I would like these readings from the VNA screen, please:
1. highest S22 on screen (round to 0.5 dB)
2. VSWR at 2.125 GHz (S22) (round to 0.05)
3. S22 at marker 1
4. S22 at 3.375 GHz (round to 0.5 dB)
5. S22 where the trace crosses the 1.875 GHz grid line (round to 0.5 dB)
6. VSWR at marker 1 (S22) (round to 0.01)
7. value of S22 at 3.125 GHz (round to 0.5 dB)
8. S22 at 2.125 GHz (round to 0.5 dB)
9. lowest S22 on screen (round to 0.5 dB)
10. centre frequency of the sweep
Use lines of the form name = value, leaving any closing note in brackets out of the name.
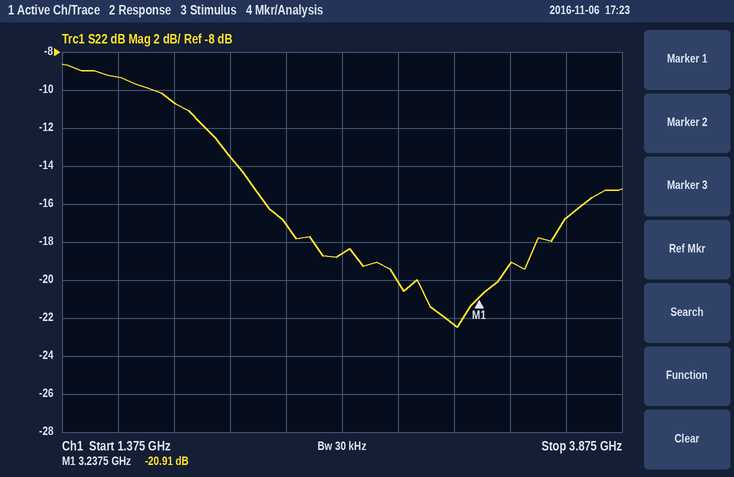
highest S22 on screen = -8.5 dB
VSWR at 2.125 GHz (S22) = 1.55
S22 at marker 1 = -20.91 dB
S22 at 3.375 GHz = -19.0 dB
S22 where the trace crosses the 1.875 GHz grid line = -10.5 dB
VSWR at marker 1 (S22) = 1.20
value of S22 at 3.125 GHz = -22.5 dB
S22 at 2.125 GHz = -13.5 dB
lowest S22 on screen = -22.5 dB
centre frequency of the sweep = 2.625 GHz
